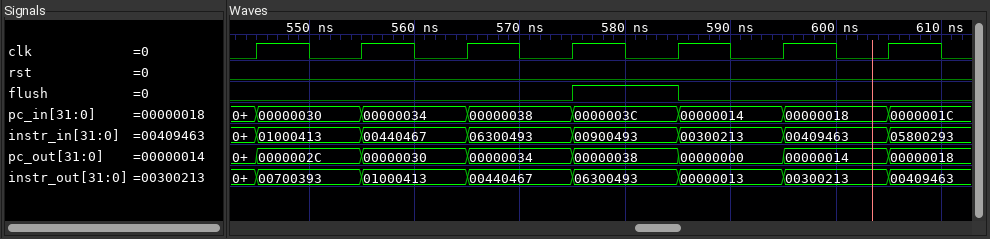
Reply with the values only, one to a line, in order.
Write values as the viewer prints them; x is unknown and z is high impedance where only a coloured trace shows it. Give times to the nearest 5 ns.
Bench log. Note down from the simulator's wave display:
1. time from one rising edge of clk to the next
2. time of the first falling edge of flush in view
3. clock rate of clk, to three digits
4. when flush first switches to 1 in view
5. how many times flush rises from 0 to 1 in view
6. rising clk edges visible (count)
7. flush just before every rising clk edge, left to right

10 ns
585 ns
100 MHz
575 ns
1
7
0 0 0 0 1 0 0
